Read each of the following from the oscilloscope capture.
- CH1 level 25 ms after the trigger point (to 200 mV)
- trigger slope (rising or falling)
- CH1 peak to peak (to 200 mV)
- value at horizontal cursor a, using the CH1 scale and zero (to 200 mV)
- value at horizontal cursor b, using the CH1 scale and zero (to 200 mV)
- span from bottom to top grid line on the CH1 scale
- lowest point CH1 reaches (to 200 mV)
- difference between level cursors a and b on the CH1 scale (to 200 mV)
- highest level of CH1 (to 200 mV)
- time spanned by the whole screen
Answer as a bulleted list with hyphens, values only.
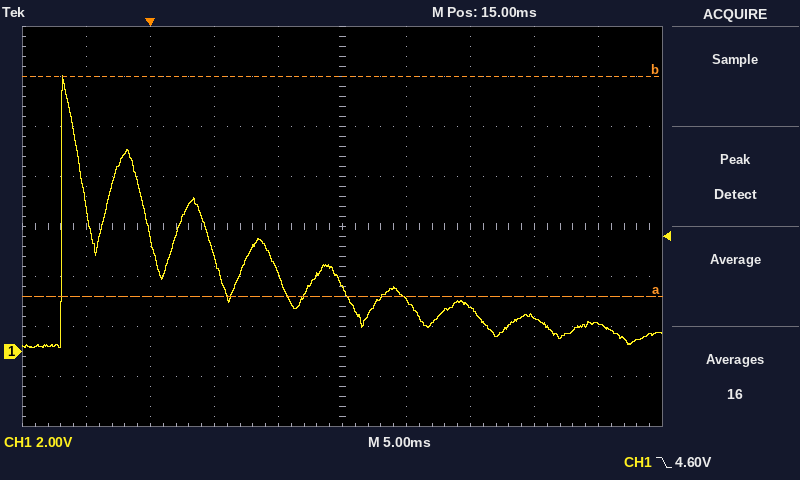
- 1.8 V
- falling
- 10.8 V
- 2.2 V
- 11.0 V
- 16 V
- 200 mV
- 8.8 V
- 11.0 V
- 50 ms
